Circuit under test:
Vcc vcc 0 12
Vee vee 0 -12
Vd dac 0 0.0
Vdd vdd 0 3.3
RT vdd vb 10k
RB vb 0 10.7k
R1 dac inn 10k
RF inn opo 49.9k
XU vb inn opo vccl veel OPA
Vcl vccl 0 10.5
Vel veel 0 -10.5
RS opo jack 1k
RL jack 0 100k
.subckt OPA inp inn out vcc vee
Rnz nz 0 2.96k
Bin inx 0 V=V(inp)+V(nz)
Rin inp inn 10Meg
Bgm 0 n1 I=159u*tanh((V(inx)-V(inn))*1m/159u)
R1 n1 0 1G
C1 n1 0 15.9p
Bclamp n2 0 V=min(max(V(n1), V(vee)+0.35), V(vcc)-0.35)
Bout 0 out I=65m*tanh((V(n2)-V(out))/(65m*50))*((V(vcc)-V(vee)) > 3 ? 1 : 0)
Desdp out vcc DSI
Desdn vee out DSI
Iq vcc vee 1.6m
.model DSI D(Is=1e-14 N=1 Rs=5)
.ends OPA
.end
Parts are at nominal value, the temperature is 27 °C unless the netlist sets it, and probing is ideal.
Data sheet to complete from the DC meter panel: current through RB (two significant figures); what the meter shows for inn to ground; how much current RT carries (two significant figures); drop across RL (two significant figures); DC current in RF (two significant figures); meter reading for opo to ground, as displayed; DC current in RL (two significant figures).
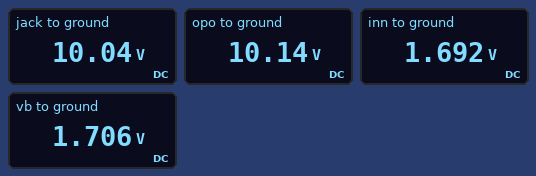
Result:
160 µA
1.692 V
160 µA
10 V
170 µA
10.14 V
100 µA
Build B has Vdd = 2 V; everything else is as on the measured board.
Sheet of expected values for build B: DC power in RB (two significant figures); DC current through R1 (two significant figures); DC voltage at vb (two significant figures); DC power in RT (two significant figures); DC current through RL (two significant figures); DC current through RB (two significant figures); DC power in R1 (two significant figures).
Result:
100 µW
100 µA
1.0 V
93 µW
61 µA
97 µA
110 µW
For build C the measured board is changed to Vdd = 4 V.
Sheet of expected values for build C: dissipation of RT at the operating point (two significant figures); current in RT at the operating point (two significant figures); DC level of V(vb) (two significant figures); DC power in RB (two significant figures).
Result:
370 µW
190 µA
2.1 V
400 µW
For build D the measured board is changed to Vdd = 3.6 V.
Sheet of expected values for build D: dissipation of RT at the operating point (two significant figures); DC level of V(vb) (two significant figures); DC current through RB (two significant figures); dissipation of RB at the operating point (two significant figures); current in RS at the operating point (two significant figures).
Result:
300 µW
1.9 V
170 µA
320 µW
100 µA
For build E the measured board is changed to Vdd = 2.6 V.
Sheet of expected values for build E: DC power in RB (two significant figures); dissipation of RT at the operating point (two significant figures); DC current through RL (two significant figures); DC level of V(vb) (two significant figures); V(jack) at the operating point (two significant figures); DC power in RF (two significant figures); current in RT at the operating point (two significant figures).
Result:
170 µW
160 µW
80 µA
1.3 V
8.0 V
900 µW
130 µA
